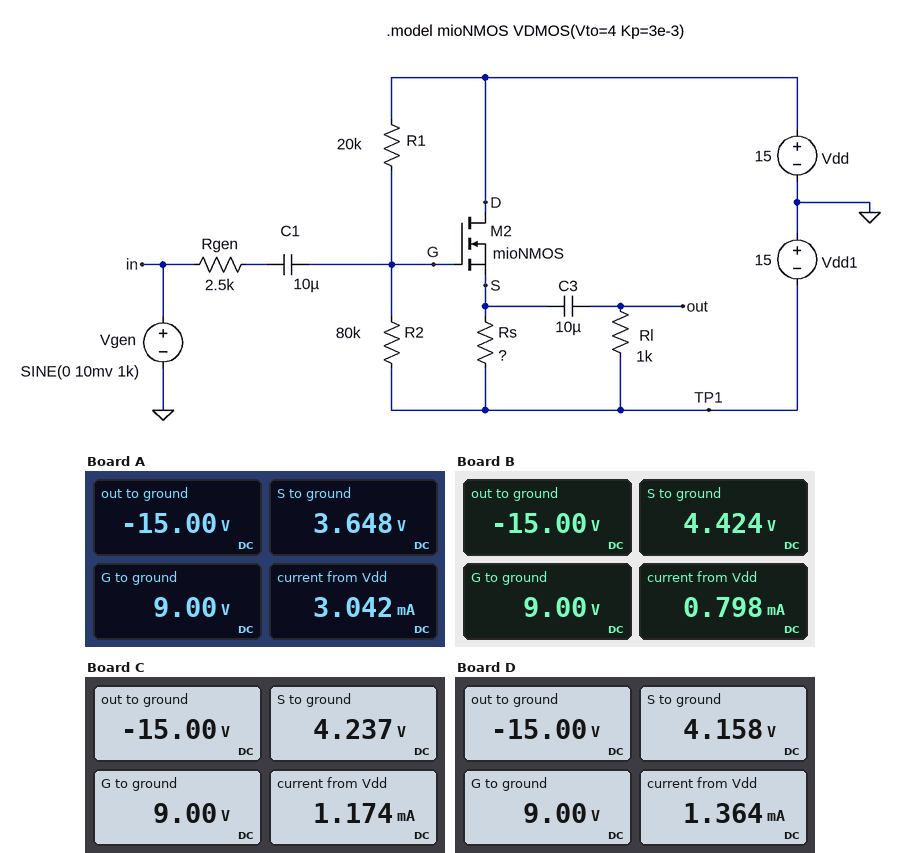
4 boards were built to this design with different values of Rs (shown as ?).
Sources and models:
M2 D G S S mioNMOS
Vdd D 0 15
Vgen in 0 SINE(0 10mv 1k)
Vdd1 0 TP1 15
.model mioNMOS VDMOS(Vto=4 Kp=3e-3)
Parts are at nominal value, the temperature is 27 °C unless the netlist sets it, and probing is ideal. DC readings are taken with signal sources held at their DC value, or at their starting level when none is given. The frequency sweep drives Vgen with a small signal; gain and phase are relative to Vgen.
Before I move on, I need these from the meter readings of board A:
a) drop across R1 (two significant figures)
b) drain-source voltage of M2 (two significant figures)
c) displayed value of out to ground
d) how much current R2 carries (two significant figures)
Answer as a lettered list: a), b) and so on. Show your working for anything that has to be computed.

a) 15 V - 9 V = 6.0 V
b) 15 V - 3.648 V = 11 V
c) -15.00 V
d) (9 V - (-15 V)) / 80 kΩ = 300 µA
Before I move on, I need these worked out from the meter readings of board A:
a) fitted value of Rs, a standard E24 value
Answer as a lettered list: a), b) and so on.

a) 6.8 kΩ
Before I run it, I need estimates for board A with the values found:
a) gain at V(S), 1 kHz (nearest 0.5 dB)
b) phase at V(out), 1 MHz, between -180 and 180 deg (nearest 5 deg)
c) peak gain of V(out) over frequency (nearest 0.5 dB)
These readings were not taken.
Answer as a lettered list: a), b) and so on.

a) -3.5 dB
b) -60 deg
c) -3.5 dB
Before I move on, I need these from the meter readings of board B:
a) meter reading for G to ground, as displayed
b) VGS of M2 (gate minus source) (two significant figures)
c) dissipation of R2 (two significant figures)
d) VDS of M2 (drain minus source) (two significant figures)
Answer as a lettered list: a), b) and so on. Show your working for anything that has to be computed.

a) 9.00 V
b) 9 V - 4.424 V = 4.6 V
c) (9 V - (-15 V))^2 / 80 kΩ = 7.2 mW
d) 15 V - 4.424 V = 11 V
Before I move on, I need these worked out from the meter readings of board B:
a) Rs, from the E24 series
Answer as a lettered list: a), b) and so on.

a) 39 kΩ
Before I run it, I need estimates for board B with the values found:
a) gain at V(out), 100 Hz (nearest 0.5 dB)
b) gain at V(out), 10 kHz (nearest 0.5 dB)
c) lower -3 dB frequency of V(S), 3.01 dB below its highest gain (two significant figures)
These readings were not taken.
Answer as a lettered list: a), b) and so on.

a) -5.5 dB
b) -5.5 dB
c) 770 mHz
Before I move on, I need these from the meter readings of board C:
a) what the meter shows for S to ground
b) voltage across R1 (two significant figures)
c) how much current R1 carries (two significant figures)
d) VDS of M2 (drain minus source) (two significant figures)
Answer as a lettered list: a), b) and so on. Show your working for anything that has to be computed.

a) 4.237 V
b) 15 V - 9 V = 6.0 V
c) (15 V - 9 V) / 20 kΩ = 300 µA
d) 15 V - 4.237 V = 11 V
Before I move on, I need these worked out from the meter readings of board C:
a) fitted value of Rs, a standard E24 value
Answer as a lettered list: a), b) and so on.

a) 22 kΩ
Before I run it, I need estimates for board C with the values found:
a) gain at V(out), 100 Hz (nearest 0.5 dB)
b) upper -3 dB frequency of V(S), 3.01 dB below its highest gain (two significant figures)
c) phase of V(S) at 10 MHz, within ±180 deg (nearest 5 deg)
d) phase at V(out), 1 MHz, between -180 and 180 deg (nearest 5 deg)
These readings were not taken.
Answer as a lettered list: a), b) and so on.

a) -4.5 dB
b) 33 kHz
c) -85 deg
d) -55 deg
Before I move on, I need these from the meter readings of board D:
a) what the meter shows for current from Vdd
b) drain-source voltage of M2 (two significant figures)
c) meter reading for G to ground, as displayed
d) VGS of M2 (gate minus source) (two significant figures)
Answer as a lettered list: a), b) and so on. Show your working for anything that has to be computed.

a) 1.364 mA
b) 15 V - 4.158 V = 11 V
c) 9.00 V
d) 9 V - 4.158 V = 4.8 V
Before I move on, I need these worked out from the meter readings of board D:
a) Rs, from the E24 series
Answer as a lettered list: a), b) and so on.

a) 18 kΩ
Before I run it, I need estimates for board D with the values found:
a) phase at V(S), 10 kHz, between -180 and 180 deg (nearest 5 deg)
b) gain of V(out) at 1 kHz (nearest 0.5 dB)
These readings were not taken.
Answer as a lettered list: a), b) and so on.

a) -5 deg
b) -4.5 dB
